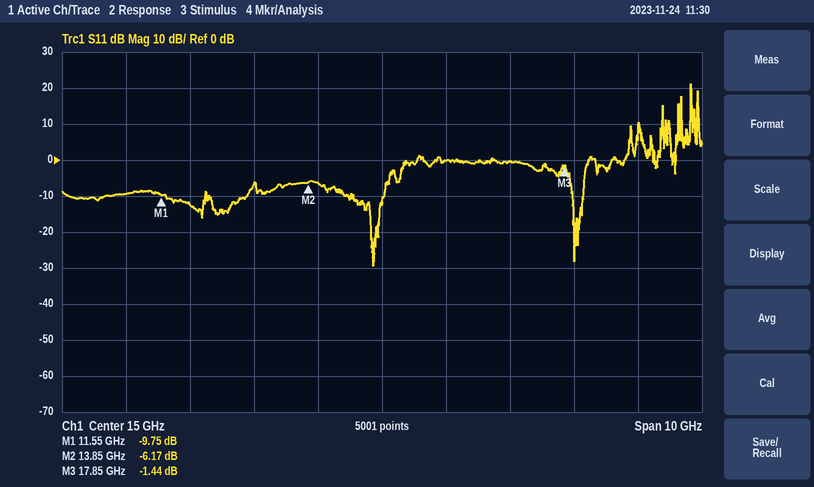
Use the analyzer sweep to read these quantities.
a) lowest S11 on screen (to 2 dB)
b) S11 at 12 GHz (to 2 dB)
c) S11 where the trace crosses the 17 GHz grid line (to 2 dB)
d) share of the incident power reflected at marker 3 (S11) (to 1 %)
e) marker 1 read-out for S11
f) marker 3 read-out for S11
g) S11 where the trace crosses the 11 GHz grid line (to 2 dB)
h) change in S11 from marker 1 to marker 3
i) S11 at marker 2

-30 dB
-12 dB
0 dB
72 %
-9.75 dB
-1.44 dB
-10 dB
8.31 dB
-6.17 dB
